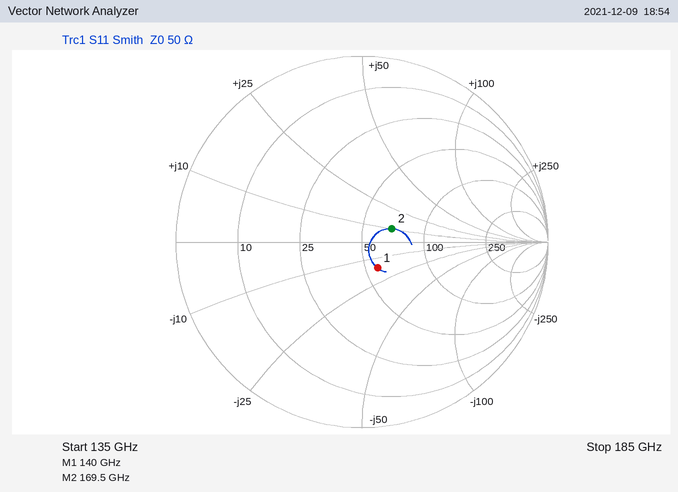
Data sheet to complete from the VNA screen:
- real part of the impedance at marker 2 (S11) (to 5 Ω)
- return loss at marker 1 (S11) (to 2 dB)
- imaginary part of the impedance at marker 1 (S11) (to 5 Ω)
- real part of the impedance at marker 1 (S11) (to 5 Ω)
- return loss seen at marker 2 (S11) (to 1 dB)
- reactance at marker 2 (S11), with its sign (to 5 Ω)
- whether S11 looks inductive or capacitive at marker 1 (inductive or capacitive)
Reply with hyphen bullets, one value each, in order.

- 70 Ω
- 16 dB
- -15 Ω
- 55 Ω
- 15 dB
- +10 Ω
- capacitive
